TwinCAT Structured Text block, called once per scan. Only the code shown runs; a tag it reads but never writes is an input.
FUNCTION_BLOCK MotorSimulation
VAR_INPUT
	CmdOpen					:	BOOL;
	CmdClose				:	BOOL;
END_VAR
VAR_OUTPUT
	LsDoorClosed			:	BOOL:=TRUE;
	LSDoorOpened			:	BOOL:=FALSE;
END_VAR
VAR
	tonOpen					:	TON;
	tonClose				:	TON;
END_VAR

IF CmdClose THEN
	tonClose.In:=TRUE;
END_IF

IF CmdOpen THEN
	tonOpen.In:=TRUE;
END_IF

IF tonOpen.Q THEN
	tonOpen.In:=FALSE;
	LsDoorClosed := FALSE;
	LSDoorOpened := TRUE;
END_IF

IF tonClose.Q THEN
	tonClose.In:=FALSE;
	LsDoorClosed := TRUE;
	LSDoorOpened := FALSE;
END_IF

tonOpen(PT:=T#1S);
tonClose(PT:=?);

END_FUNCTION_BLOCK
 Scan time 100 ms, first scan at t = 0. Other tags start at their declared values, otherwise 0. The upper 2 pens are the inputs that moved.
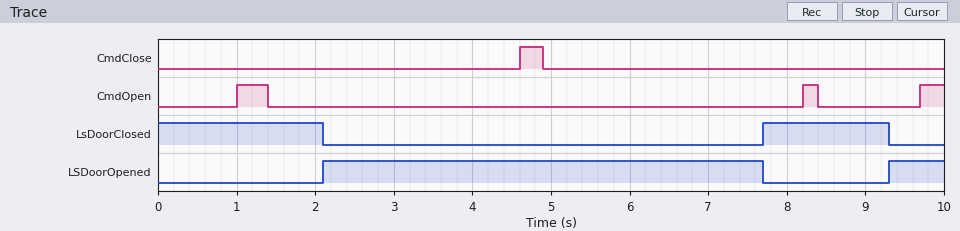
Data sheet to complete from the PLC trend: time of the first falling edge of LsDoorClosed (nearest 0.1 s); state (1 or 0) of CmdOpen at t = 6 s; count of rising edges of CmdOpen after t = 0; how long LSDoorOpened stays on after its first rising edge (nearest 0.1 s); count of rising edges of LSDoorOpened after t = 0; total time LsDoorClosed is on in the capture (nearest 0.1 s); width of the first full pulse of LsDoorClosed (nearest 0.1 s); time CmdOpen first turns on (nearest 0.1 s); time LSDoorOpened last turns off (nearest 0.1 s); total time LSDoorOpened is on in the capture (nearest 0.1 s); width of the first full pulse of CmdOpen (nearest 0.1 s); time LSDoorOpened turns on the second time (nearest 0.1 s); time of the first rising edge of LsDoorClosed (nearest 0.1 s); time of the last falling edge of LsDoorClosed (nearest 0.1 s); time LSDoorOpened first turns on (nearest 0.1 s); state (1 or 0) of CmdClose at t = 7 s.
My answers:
2.1 s
0
3
5.6 s
2
3.7 s
1.6 s
1.0 s
7.7 s
6.3 s
0.4 s
9.3 s
7.7 s
9.3 s
2.1 s
0
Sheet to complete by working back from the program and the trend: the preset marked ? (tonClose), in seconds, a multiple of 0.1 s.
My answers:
3.0 s
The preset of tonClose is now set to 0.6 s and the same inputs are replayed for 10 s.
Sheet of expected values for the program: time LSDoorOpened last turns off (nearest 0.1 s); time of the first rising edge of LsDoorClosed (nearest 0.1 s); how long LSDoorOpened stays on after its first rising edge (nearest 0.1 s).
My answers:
5.3 s
5.3 s
3.2 s
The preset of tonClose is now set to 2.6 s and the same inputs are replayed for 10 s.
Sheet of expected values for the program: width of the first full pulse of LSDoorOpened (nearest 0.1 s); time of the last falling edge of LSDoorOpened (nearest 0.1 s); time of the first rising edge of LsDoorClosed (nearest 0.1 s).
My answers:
5.2 s
7.3 s
7.3 s
